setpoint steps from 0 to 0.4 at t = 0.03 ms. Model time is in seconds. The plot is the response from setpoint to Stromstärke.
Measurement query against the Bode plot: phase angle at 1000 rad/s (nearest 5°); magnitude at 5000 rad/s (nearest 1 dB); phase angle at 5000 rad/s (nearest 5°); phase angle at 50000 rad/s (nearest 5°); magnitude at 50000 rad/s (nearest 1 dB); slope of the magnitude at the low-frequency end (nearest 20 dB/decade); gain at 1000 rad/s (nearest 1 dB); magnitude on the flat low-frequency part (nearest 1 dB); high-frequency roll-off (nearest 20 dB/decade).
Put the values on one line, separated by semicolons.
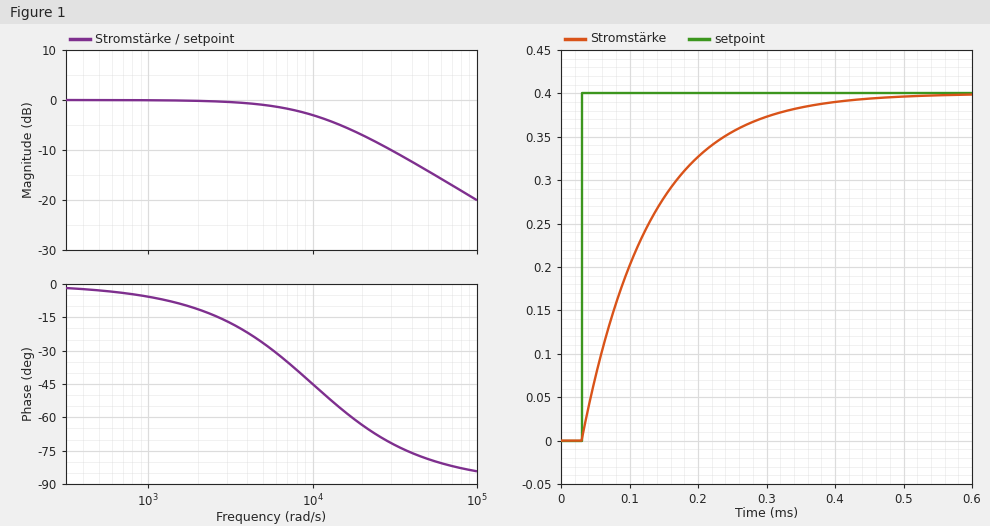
-5°; -1 dB; -25°; -80°; -14 dB; 0 dB/decade; 0 dB; 0 dB; -20 dB/decade
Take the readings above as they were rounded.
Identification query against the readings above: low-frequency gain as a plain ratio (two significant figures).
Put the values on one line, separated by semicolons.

1.0
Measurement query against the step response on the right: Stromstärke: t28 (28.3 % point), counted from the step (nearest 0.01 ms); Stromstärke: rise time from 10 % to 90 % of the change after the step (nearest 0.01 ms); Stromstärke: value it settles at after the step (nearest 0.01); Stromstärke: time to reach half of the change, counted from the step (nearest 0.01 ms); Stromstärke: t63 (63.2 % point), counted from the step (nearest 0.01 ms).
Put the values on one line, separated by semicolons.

0.03 ms; 0.22 ms; 0.40; 0.07 ms; 0.10 ms
